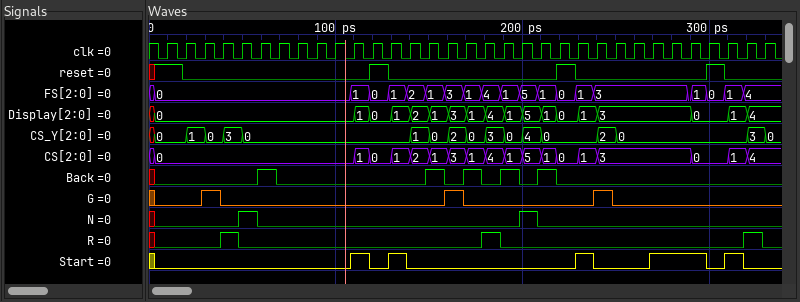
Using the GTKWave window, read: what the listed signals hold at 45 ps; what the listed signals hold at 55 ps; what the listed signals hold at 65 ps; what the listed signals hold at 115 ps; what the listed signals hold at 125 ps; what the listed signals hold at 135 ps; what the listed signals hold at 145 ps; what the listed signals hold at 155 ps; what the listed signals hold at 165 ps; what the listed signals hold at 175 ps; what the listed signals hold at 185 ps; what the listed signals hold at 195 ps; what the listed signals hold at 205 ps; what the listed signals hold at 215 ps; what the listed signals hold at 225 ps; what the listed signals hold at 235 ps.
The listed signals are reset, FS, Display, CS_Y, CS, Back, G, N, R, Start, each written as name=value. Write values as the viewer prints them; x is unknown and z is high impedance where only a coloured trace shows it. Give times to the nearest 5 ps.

reset=0, FS=0, Display=0, CS_Y=3, CS=0, Back=0, G=0, N=0, R=1, Start=0
reset=0, FS=0, Display=0, CS_Y=0, CS=0, Back=0, G=0, N=1, R=0, Start=0
reset=0, FS=0, Display=0, CS_Y=0, CS=0, Back=1, G=0, N=0, R=0, Start=0
reset=0, FS=1, Display=1, CS_Y=0, CS=1, Back=0, G=0, N=0, R=0, Start=1
reset=1, FS=0, Display=0, CS_Y=0, CS=0, Back=0, G=0, N=0, R=0, Start=0
reset=0, FS=1, Display=1, CS_Y=0, CS=1, Back=0, G=0, N=0, R=0, Start=1
reset=0, FS=2, Display=2, CS_Y=1, CS=2, Back=0, G=0, N=0, R=0, Start=0
reset=0, FS=1, Display=1, CS_Y=0, CS=1, Back=1, G=0, N=0, R=0, Start=0
reset=0, FS=3, Display=3, CS_Y=2, CS=3, Back=0, G=1, N=0, R=0, Start=0
reset=0, FS=1, Display=1, CS_Y=0, CS=1, Back=1, G=0, N=0, R=0, Start=0
reset=0, FS=4, Display=4, CS_Y=3, CS=4, Back=0, G=0, N=0, R=1, Start=0
reset=0, FS=1, Display=1, CS_Y=0, CS=1, Back=1, G=0, N=0, R=0, Start=0
reset=0, FS=5, Display=5, CS_Y=4, CS=5, Back=0, G=0, N=1, R=0, Start=0
reset=0, FS=1, Display=1, CS_Y=0, CS=1, Back=1, G=0, N=0, R=0, Start=0
reset=1, FS=0, Display=0, CS_Y=0, CS=0, Back=0, G=0, N=0, R=0, Start=0
reset=0, FS=1, Display=1, CS_Y=0, CS=1, Back=0, G=0, N=0, R=0, Start=1
